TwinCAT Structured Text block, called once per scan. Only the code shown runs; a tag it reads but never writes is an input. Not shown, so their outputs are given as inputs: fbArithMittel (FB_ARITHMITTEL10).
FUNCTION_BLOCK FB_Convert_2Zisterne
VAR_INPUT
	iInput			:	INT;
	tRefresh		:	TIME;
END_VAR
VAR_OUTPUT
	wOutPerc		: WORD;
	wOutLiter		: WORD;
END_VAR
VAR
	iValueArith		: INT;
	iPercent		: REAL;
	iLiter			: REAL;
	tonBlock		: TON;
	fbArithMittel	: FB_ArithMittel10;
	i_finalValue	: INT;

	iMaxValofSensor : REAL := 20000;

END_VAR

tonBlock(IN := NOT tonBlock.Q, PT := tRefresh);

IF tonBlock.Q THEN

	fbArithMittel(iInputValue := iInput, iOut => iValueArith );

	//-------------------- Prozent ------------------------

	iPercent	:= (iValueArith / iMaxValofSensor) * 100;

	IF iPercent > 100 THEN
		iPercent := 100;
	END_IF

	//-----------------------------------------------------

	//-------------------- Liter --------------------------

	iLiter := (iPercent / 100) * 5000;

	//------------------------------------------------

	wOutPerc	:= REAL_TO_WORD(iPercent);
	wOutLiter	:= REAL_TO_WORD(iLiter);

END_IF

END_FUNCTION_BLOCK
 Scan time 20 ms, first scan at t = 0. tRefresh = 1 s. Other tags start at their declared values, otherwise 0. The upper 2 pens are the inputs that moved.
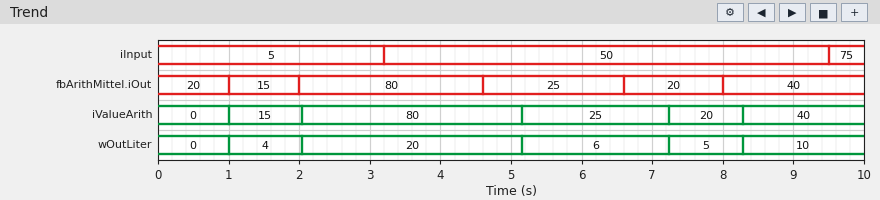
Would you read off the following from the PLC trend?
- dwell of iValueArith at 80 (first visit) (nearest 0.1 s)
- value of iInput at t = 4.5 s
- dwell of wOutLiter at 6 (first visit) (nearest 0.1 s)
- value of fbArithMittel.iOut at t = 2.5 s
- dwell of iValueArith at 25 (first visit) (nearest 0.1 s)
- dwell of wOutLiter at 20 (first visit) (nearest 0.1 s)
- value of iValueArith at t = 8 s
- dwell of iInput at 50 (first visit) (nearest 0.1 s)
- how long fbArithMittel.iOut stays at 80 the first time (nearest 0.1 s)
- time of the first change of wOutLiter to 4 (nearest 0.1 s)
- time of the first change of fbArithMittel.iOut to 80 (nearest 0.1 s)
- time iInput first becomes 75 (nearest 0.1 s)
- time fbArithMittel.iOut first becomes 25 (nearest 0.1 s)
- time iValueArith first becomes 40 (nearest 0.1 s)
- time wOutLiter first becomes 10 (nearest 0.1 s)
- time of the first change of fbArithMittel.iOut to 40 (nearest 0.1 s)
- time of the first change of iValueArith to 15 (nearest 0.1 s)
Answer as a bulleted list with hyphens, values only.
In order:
- 3.1 s
- 50
- 2.1 s
- 80
- 2.1 s
- 3.1 s
- 20
- 6.3 s
- 2.6 s
- 1.0 s
- 2.0 s
- 9.5 s
- 4.6 s
- 8.3 s
- 8.3 s
- 8.0 s
- 1.0 s
